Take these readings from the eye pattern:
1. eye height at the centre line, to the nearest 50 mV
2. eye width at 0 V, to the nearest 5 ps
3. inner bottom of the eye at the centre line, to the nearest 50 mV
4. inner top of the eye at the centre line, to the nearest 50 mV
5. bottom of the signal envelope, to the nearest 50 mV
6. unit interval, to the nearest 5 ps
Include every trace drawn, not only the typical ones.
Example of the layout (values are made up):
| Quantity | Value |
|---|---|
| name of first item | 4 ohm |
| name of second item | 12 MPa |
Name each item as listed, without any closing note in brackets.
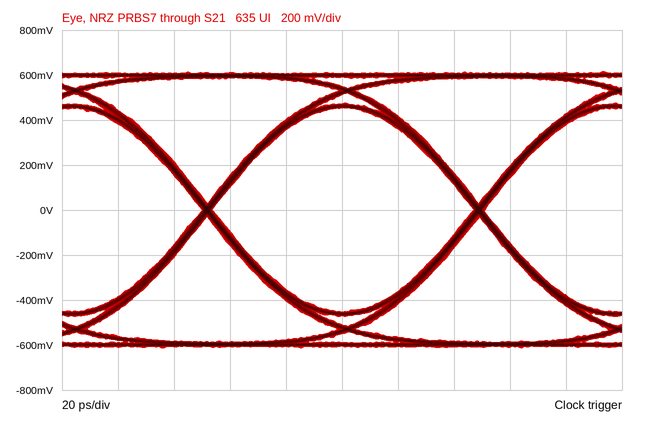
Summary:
| Quantity | Value |
|---|---|
| eye height at the centre line, to the nearest 50 mV | 900 mV |
| eye width at 0 V, to the nearest 5 ps | 95 ps |
| inner bottom of the eye at the centre line, to the nearest 50 mV | -450 mV |
| inner top of the eye at the centre line, to the nearest 50 mV | 450 mV |
| bottom of the signal envelope, to the nearest 50 mV | -600 mV |
| unit interval, to the nearest 5 ps | 95 ps |
